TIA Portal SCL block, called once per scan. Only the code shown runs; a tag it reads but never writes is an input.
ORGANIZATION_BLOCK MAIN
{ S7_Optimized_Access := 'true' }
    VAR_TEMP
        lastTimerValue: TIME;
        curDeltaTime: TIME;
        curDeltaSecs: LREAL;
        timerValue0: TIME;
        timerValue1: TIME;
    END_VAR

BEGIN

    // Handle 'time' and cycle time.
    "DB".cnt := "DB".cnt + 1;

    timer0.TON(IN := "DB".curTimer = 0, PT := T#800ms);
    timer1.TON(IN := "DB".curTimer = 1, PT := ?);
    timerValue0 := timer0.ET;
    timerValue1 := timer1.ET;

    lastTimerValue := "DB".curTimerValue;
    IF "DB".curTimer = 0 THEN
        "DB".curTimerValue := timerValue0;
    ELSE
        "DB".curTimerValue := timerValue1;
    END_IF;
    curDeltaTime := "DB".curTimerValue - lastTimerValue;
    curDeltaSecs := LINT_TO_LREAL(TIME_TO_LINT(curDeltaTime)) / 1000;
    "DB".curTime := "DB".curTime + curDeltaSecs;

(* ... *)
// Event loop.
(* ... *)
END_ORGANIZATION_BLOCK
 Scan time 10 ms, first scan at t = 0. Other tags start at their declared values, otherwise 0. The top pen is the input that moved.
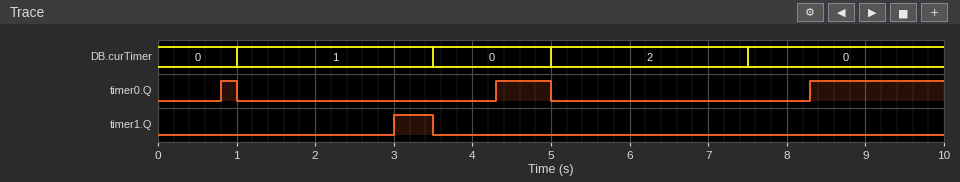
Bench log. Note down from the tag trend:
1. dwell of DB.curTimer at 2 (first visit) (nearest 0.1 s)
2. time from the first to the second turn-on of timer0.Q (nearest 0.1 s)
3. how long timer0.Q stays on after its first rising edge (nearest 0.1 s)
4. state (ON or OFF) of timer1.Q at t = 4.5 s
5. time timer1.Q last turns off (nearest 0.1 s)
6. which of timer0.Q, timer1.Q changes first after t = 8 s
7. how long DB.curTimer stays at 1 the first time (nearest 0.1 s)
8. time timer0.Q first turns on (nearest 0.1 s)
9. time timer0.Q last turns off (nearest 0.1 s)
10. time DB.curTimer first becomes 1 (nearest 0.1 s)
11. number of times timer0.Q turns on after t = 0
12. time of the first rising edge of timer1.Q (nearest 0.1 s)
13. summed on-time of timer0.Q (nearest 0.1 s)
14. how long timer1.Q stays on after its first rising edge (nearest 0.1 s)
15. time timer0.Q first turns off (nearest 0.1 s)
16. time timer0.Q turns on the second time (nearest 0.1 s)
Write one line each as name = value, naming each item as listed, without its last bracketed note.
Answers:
dwell of DB.curTimer at 2 (first visit) = 2.5 s
time from the first to the second turn-on of timer0.Q = 3.5 s
how long timer0.Q stays on after its first rising edge = 0.2 s
state (ON or OFF) of timer1.Q at t = 4.5 s = OFF
time timer1.Q last turns off = 3.5 s
which of timer0.Q, timer1.Q changes first after t = 8 s = timer0.Q
how long DB.curTimer stays at 1 the first time = 2.5 s
time timer0.Q first turns on = 0.8 s
time timer0.Q last turns off = 5.0 s
time DB.curTimer first becomes 1 = 1.0 s
number of times timer0.Q turns on after t = 0 = 3
time of the first rising edge of timer1.Q = 3.0 s
summed on-time of timer0.Q = 2.6 s
how long timer1.Q stays on after its first rising edge = 0.5 s
time timer0.Q first turns off = 1.0 s
time timer0.Q turns on the second time = 4.3 s
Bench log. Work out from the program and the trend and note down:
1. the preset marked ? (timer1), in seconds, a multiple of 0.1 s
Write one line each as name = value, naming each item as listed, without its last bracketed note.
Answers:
the preset marked ? (timer1), in seconds, a multiple of 0.1 s = 2.0 s
